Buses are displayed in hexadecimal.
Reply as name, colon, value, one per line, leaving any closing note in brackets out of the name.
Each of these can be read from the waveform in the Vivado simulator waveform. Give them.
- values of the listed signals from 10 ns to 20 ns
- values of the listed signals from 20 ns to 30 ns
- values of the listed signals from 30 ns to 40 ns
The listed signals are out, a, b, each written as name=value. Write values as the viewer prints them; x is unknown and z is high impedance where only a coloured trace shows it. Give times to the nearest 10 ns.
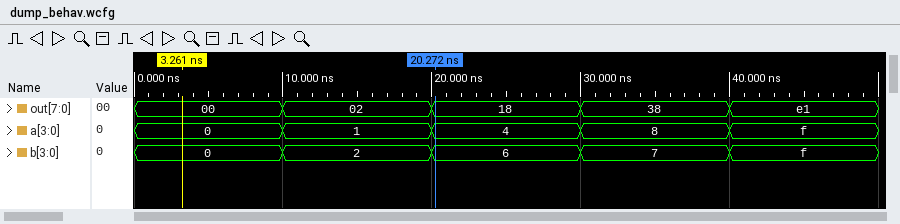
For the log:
values of the listed signals from 10 ns to 20 ns: out=02, a=1, b=2
values of the listed signals from 20 ns to 30 ns: out=18, a=4, b=6
values of the listed signals from 30 ns to 40 ns: out=38, a=8, b=7
